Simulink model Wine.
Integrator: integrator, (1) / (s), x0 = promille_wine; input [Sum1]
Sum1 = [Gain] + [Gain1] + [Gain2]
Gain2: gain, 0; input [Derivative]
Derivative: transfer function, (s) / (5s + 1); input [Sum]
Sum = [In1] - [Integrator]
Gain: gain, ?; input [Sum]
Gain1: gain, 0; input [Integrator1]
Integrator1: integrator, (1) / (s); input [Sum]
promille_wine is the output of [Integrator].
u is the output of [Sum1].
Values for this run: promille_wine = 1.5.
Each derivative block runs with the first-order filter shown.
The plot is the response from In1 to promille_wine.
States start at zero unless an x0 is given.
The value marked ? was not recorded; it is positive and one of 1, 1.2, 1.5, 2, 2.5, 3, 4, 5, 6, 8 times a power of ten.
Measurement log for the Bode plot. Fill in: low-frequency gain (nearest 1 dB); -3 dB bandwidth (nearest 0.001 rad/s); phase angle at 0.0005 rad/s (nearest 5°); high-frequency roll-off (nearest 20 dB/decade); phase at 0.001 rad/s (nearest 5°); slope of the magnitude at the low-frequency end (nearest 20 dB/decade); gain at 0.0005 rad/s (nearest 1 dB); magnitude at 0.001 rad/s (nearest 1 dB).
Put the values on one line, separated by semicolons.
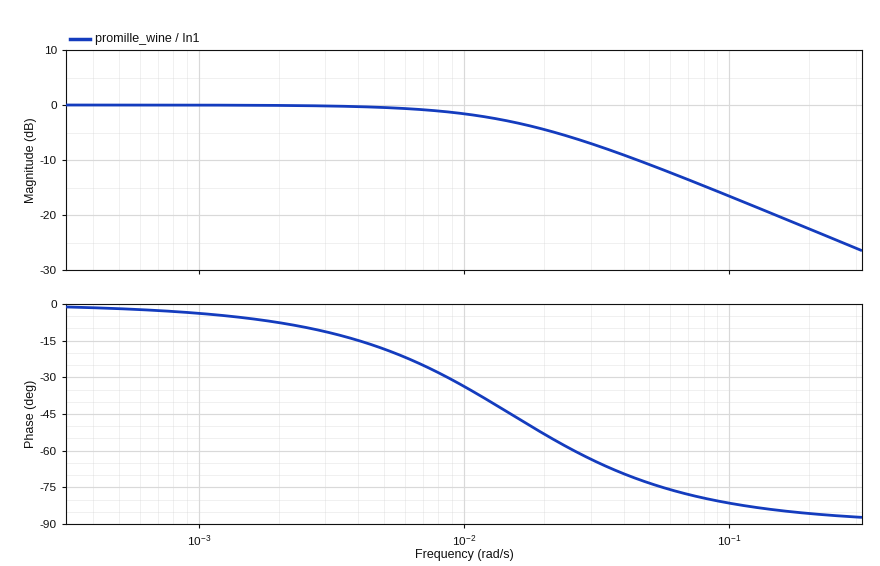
0 dB; 0.015 rad/s; 0°; -20 dB/decade; -5°; 0 dB/decade; 0 dB; 0 dB
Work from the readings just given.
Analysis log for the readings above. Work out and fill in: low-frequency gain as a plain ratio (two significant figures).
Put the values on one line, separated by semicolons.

1.0
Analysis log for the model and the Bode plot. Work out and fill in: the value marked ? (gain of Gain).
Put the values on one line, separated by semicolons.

0.015
